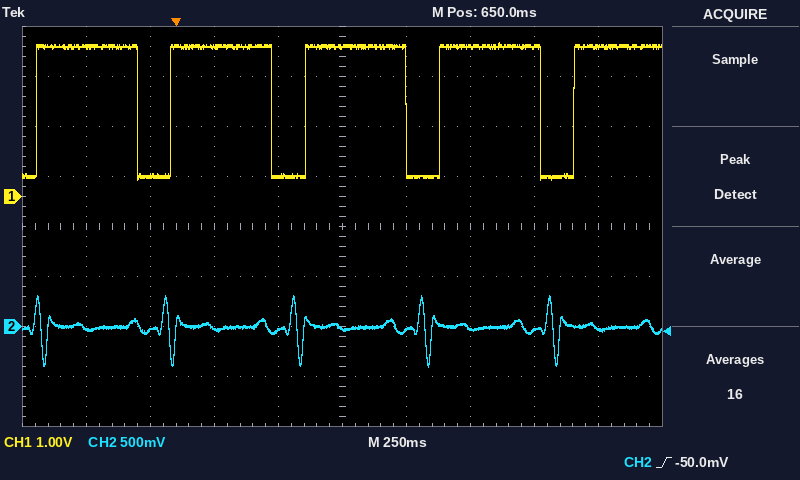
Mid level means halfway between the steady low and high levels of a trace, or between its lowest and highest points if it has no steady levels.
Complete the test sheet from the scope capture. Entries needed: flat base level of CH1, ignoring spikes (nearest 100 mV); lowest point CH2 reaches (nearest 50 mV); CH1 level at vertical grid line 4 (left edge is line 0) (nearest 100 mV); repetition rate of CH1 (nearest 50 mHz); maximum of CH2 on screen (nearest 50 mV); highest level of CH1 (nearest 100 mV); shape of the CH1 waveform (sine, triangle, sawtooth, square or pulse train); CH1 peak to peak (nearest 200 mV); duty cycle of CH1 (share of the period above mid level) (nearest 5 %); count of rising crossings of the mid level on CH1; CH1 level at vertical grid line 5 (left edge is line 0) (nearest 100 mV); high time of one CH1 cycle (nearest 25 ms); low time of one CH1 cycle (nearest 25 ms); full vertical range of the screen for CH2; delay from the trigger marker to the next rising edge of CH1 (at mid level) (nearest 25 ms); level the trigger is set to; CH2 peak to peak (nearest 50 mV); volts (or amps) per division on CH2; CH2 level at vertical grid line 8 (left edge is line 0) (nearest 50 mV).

400 mV
-400 mV
400 mV
1.90 Hz
300 mV
3.1 V
pulse train
2.8 V
75 %
5
3.0 V
400 ms
125 ms
4 V
500 ms
-50.0 mV
700 mV
500 mV
-50 mV
